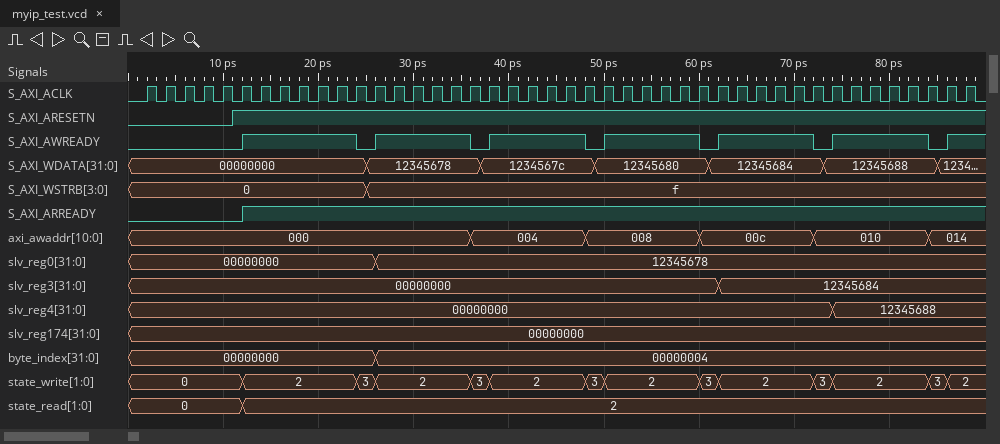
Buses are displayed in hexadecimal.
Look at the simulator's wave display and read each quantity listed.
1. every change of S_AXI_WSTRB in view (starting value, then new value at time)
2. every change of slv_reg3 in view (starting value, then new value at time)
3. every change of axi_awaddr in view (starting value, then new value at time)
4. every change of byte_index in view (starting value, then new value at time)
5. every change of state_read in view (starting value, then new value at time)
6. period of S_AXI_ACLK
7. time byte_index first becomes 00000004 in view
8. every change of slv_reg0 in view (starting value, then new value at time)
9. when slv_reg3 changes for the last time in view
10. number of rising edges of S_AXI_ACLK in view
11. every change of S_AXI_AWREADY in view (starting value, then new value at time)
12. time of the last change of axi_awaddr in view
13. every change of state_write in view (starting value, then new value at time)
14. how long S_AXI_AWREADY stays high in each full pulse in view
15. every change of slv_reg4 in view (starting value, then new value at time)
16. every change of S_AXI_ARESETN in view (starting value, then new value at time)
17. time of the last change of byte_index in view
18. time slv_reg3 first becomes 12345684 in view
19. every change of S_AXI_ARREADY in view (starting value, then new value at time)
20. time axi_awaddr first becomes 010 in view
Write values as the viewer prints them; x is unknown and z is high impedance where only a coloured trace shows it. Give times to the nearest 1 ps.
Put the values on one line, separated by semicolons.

0, f at 25 ps; 00000000, 12345684 at 62 ps; 000, 004 at 36 ps, 008 at 48 ps, 00c at 60 ps, 010 at 72 ps, 014 at 84 ps; 00000000, 00000004 at 26 ps; 0, 2 at 12 ps; 2 ps; 26 ps; 00000000, 12345678 at 26 ps; 62 ps; 44; 0, 1 at 12 ps, 0 at 24 ps, 1 at 26 ps, 0 at 36 ps, 1 at 38 ps, 0 at 48 ps, 1 at 50 ps, 0 at 60 ps, 1 at 62 ps, 0 at 72 ps, 1 at 74 ps, 0 at 84 ps, 1 at 86 ps; 84 ps; 0, 2 at 12 ps, 3 at 24 ps, 2 at 26 ps, 3 at 36 ps, 2 at 38 ps, 3 at 48 ps, 2 at 50 ps, 3 at 60 ps, 2 at 62 ps, 3 at 72 ps, 2 at 74 ps, 3 at 84 ps, 2 at 86 ps; 12 ps, 10 ps, 10 ps, 10 ps, 10 ps, 10 ps; 00000000, 12345688 at 74 ps; 0, 1 at 11 ps; 26 ps; 62 ps; 0, 1 at 12 ps; 72 ps
